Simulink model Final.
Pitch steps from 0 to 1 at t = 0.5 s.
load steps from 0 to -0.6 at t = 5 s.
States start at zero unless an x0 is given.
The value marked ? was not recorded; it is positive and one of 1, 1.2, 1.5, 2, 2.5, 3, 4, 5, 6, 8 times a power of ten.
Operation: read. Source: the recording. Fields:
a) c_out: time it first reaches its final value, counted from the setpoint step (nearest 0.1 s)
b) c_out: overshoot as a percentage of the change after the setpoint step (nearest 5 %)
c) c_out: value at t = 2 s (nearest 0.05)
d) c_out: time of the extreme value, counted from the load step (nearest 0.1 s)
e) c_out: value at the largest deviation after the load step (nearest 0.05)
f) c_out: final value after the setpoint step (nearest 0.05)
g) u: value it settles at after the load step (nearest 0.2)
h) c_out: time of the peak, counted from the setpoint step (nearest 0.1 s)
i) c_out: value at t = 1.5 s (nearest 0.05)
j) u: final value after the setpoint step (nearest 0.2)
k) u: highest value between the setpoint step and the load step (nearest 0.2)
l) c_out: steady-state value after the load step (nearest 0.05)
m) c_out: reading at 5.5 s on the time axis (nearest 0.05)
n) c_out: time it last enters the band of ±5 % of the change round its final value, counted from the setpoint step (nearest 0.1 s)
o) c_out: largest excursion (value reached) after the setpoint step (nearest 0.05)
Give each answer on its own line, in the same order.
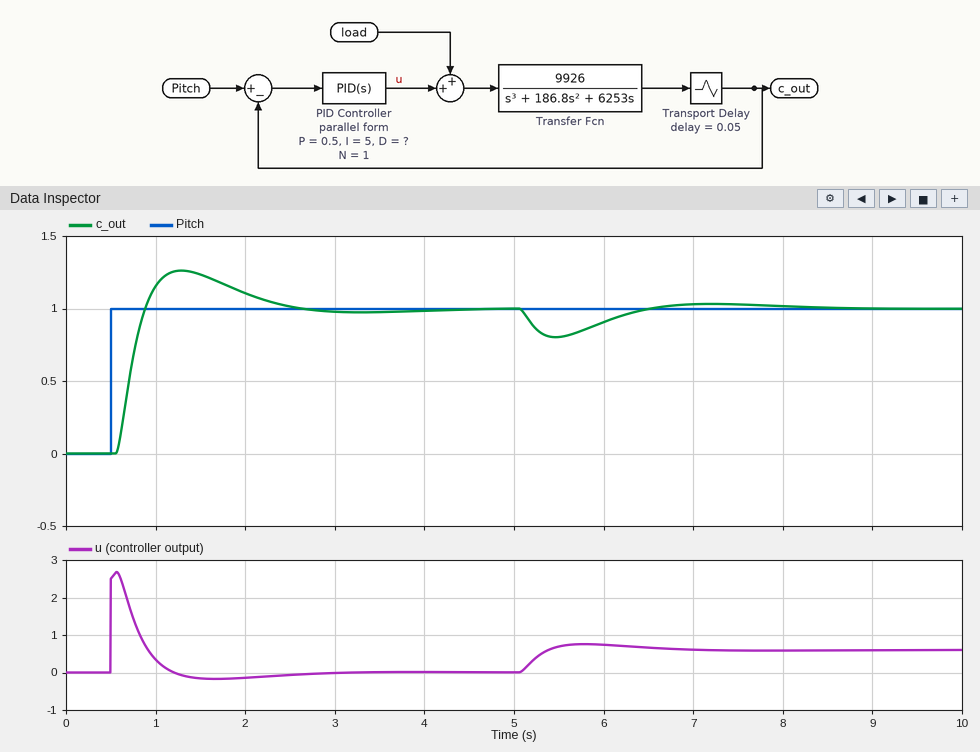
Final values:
0.4 s
25 %
1.10
0.5 s
0.80
1.00
0.6
0.8 s
1.25
0.0
2.6
1.00
0.80
1.8 s
1.25
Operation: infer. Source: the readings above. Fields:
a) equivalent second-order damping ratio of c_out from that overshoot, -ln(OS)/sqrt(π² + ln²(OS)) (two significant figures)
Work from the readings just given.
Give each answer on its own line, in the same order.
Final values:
0.40
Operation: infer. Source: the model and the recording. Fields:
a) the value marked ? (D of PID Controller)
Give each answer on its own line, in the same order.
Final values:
2
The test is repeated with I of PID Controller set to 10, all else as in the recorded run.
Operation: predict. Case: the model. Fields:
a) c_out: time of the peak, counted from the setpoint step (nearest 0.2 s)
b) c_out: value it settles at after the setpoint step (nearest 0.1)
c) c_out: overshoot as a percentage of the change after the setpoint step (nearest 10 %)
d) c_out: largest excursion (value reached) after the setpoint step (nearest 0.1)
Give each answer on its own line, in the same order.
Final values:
0.6 s
1.0
50 %
1.5
